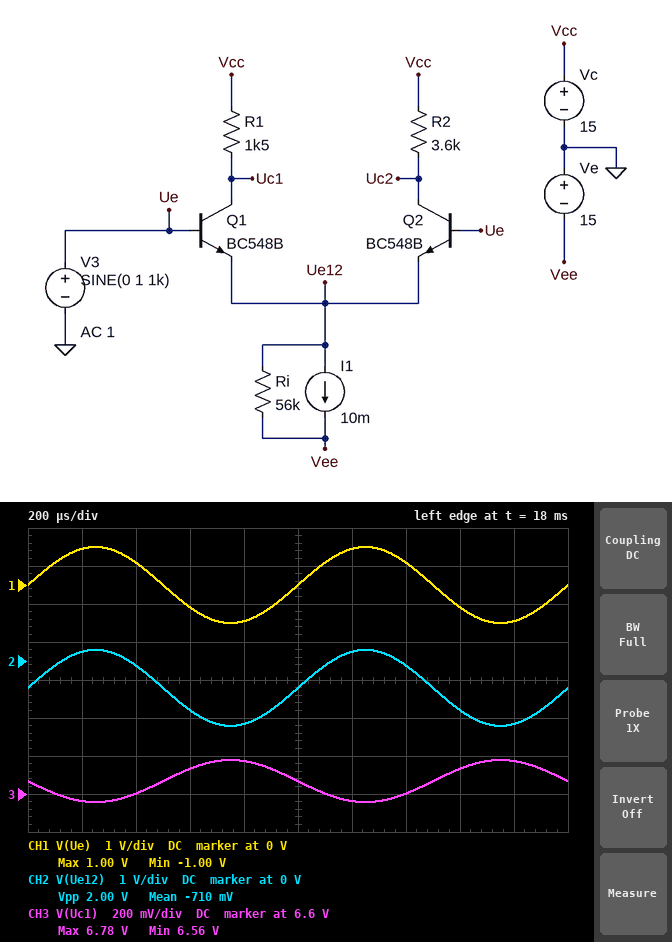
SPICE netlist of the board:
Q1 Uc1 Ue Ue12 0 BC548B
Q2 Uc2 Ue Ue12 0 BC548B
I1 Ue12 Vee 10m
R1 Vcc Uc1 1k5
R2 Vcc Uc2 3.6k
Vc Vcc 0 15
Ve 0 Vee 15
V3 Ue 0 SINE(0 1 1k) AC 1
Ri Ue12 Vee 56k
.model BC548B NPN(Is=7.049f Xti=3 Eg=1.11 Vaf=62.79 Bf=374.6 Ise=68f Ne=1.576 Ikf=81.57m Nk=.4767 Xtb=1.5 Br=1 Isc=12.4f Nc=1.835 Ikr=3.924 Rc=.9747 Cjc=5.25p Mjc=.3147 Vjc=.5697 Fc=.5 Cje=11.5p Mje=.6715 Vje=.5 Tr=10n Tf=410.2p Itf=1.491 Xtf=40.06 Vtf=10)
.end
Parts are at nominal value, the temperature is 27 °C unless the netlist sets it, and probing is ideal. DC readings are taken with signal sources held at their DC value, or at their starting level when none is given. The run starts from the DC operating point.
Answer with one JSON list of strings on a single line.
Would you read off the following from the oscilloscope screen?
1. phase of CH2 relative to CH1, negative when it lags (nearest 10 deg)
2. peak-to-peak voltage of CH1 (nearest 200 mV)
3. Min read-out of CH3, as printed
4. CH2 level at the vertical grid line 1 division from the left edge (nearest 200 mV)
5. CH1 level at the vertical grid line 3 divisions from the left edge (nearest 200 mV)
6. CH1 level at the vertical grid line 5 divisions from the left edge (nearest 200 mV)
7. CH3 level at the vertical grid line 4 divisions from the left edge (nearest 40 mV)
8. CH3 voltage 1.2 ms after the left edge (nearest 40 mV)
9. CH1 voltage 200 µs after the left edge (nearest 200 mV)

["0 deg", "2.0 V", "6.56 V", "200 mV", "-600 mV", "0 V", "6.76 V", "6.56 V", "1.0 V"]
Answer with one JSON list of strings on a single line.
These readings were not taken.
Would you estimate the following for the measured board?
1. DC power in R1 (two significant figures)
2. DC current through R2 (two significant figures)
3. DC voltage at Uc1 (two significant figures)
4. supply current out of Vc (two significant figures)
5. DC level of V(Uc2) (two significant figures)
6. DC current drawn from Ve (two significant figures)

["46 mW", "4.3 mA", "6.7 V", "9.9 mA", "-630 mV", "10 mA"]
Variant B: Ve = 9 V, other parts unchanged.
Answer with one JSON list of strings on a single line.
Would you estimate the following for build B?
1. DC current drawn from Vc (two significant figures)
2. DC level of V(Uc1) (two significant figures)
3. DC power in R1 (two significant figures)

["9.8 mA", "6.8 V", "45 mW"]
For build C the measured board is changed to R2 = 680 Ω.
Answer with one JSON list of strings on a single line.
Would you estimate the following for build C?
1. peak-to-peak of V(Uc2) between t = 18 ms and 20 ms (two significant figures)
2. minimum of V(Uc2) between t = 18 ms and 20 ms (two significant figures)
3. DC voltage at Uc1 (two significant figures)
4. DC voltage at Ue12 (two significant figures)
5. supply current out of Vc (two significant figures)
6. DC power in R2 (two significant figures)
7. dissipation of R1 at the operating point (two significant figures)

["15 mV", "11 V", "7.5 V", "-700 mV", "10 mA", "19 mW", "37 mW"]
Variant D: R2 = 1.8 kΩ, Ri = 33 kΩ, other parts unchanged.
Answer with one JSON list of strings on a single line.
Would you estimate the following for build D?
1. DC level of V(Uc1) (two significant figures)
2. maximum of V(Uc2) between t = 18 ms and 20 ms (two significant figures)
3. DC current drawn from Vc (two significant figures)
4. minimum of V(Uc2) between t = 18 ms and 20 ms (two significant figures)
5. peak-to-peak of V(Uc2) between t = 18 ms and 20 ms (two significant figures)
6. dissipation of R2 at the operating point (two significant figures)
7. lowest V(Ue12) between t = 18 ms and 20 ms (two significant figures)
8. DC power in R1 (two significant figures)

["7.1 V", "5.8 V", "10 mA", "5.7 V", "50 mV", "48 mW", "-1.7 V", "41 mW"]
